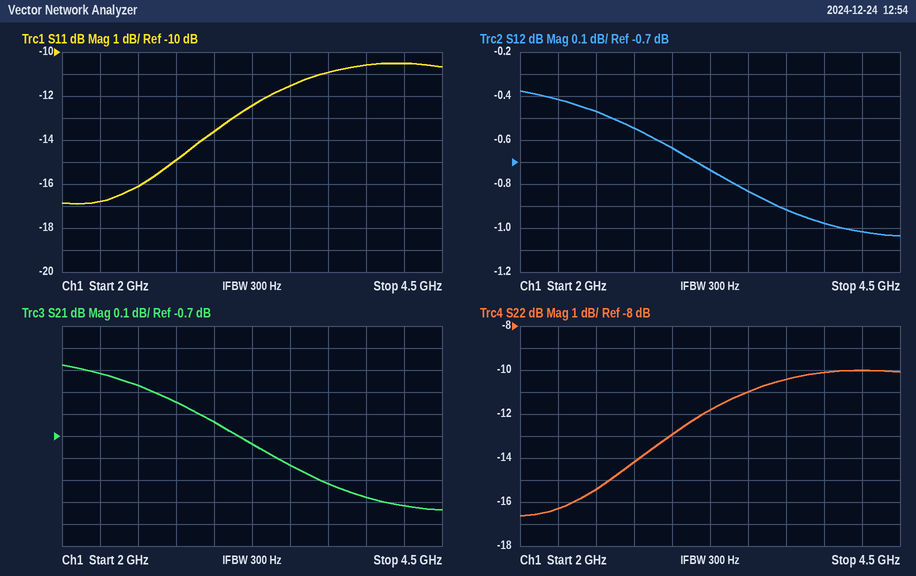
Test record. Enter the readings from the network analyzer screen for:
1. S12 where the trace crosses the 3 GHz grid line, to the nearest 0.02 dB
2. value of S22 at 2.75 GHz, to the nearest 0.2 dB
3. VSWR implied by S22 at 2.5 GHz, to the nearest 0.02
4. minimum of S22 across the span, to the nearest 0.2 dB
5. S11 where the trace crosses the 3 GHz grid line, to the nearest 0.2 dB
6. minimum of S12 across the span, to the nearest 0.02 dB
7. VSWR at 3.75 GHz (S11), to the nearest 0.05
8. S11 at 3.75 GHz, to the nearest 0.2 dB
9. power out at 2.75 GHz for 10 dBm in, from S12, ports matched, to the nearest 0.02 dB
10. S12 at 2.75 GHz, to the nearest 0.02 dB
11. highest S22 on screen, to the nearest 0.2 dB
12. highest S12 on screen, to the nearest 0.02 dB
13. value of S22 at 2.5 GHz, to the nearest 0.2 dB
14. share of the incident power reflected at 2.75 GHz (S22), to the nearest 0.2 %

-0.64 dB
-14.2 dB
1.40
-16.6 dB
-13.6 dB
-1.04 dB
1.80
-11.0 dB
9.46 dBm
-0.54 dB
-10.0 dB
-0.38 dB
-15.4 dB
3.8 %
